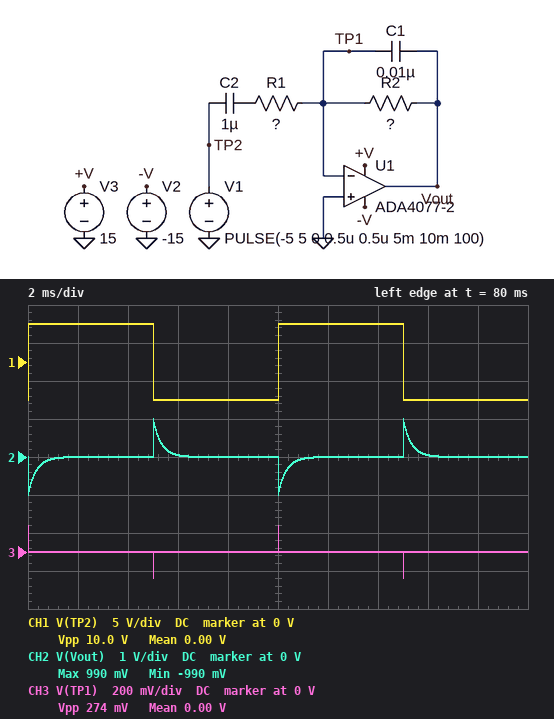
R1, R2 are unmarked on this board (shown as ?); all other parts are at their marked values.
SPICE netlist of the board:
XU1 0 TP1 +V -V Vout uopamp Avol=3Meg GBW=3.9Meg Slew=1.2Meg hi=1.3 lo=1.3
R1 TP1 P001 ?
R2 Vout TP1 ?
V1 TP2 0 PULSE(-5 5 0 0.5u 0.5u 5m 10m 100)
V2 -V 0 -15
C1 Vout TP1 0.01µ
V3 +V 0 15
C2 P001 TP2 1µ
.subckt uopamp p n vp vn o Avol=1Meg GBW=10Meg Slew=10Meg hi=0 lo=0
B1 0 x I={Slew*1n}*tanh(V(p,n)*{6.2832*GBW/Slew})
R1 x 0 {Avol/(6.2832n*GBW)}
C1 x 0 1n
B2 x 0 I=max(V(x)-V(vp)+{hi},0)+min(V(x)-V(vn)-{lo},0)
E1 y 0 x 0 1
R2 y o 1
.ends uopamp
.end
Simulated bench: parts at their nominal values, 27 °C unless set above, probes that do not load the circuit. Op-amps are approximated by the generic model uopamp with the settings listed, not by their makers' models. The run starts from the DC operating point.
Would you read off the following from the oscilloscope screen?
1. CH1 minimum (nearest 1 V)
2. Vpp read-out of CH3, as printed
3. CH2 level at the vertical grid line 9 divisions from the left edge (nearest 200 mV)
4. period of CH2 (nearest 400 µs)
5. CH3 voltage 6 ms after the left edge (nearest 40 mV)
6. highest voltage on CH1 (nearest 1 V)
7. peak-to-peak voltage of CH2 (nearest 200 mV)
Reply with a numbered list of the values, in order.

1. -5 V
2. 274 mV
3. 0 V
4. 10.0 ms
5. 0 V
6. 5 V
7. 2.0 V
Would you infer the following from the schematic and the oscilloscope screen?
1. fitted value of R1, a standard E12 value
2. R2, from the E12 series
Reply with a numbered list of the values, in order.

1. 330 Ω
2. 33 Ω
